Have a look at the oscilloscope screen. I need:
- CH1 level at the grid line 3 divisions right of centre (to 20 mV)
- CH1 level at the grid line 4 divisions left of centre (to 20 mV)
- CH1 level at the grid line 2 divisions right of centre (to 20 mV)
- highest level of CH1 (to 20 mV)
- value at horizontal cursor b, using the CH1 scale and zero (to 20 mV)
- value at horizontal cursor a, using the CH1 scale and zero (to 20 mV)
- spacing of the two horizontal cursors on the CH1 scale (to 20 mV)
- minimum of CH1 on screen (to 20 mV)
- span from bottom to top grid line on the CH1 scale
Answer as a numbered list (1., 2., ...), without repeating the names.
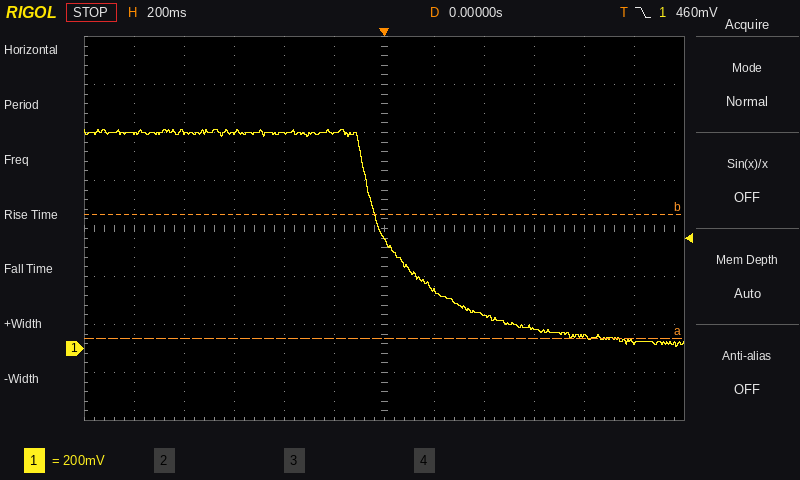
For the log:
1. 80 mV
2. 900 mV
3. 140 mV
4. 920 mV
5. 560 mV
6. 40 mV
7. 520 mV
8. 0 mV
9. 1.6 V
